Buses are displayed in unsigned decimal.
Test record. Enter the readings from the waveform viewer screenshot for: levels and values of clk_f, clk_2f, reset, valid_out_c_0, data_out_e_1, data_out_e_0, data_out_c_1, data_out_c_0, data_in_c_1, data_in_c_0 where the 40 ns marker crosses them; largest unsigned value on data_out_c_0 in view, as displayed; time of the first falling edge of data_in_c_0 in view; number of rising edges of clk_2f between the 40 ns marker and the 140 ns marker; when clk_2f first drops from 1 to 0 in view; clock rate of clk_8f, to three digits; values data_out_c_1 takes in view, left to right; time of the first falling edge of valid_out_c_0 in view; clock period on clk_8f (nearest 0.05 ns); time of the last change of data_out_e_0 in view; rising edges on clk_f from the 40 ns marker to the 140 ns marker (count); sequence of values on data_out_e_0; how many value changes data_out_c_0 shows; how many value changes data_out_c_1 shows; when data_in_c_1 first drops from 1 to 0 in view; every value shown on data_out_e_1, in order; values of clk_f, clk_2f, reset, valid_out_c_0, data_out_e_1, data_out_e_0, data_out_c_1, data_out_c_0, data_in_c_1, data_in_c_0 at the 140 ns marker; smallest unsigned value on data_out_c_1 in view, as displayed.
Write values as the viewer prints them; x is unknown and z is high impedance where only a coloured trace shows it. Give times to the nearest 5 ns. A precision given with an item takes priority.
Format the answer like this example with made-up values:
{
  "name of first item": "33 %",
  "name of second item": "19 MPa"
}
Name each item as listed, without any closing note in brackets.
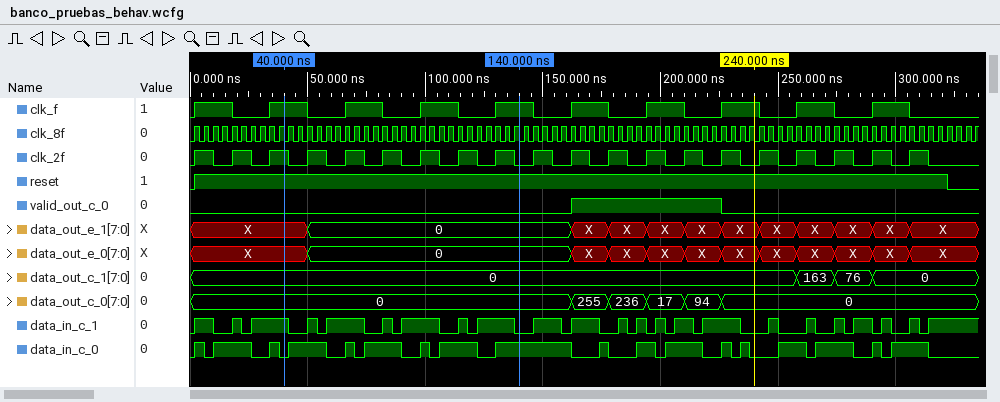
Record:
{
  "levels and values of clk_f, clk_2f, reset, valid_out_c_0, data_out_e_1, data_out_e_0, data_out_c_1, data_out_c_0, data_in_c_1, data_in_c_0 where the 40 ns marker crosses them": "clk_f=1, clk_2f=1, reset=1, valid_out_c_0=0, data_out_e_1=X, data_out_e_0=X, data_out_c_1=0, data_out_c_0=0, data_in_c_1=1, data_in_c_0=0",
  "largest unsigned value on data_out_c_0 in view, as displayed": "255",
  "time of the first falling edge of data_in_c_0 in view": "5 ns",
  "number of rising edges of clk_2f between the 40 ns marker and the 140 ns marker": "6",
  "when clk_2f first drops from 1 to 0 in view": "10 ns",
  "clock rate of clk_8f, to three digits": "250 MHz",
  "values data_out_c_1 takes in view, left to right": "0, 163, 76, 0",
  "time of the first falling edge of valid_out_c_0 in view": "225 ns",
  "clock period on clk_8f": "4 ns",
  "time of the last change of data_out_e_0 in view": "305 ns",
  "rising edges on clk_f from the 40 ns marker to the 140 ns marker": "3",
  "sequence of values on data_out_e_0": "X, 0, X, X, X, X, X, X, X, X, X, X",
  "how many value changes data_out_c_0 shows": "5",
  "how many value changes data_out_c_1 shows": "3",
  "when data_in_c_1 first drops from 1 to 0 in view": "10 ns",
  "every value shown on data_out_e_1, in order": "X, 0, X, X, X, X, X, X, X, X, X, X",
  "values of clk_f, clk_2f, reset, valid_out_c_0, data_out_e_1, data_out_e_0, data_out_c_1, data_out_c_0, data_in_c_1, data_in_c_0 at the 140 ns marker": "clk_f=1, clk_2f=0, reset=1, valid_out_c_0=0, data_out_e_1=0, data_out_e_0=0, data_out_c_1=0, data_out_c_0=0, data_in_c_1=0, data_in_c_0=1",
  "smallest unsigned value on data_out_c_1 in view, as displayed": "0"
}
